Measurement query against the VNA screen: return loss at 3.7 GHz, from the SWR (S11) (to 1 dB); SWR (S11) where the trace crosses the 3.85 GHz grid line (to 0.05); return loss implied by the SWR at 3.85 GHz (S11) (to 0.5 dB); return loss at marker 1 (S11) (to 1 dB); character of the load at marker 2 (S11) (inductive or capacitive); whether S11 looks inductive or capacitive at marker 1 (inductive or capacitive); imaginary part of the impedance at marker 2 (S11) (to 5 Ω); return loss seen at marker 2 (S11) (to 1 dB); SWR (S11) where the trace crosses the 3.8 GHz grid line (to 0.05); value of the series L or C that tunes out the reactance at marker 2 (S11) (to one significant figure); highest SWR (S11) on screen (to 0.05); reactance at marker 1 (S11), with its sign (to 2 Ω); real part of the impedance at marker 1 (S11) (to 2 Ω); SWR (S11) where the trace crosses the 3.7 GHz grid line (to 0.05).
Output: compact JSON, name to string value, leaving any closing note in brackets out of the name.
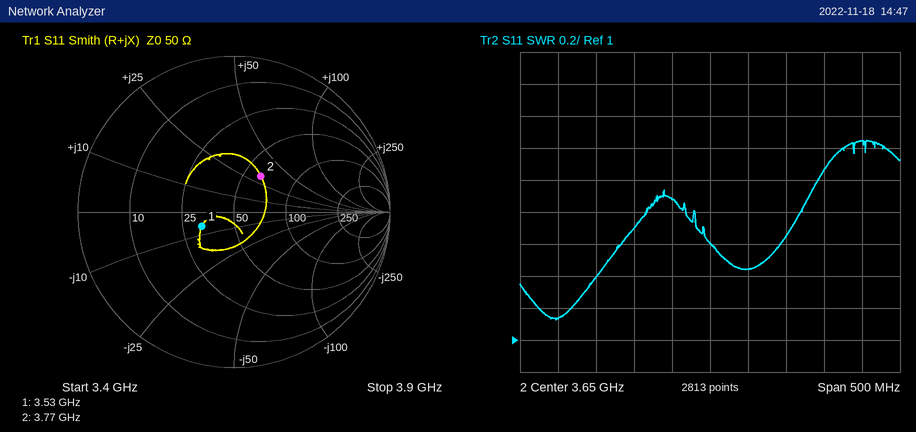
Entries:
{"return loss at 3.7 GHz, from the SWR (S11)": "15 dB", "SWR (S11) where the trace crosses the 3.85 GHz grid line": "2.25", "return loss implied by the SWR at 3.85 GHz (S11)": "8.5 dB", "return loss at marker 1 (S11)": "13 dB", "character of the load at marker 2 (S11)": "inductive", "whether S11 looks inductive or capacitive at marker 1": "capacitive", "imaginary part of the impedance at marker 2 (S11)": "+30 Ω", "return loss seen at marker 2 (S11)": "11 dB", "SWR (S11) where the trace crosses the 3.8 GHz grid line": "2.05", "value of the series L or C that tunes out the reactance at marker 2 (S11)": "1 pF", "highest SWR (S11) on screen": "2.25", "reactance at marker 1 (S11), with its sign": "-6 Ω", "real part of the impedance at marker 1 (S11)": "32 Ω", "SWR (S11) where the trace crosses the 3.7 GHz grid line": "1.45"}
